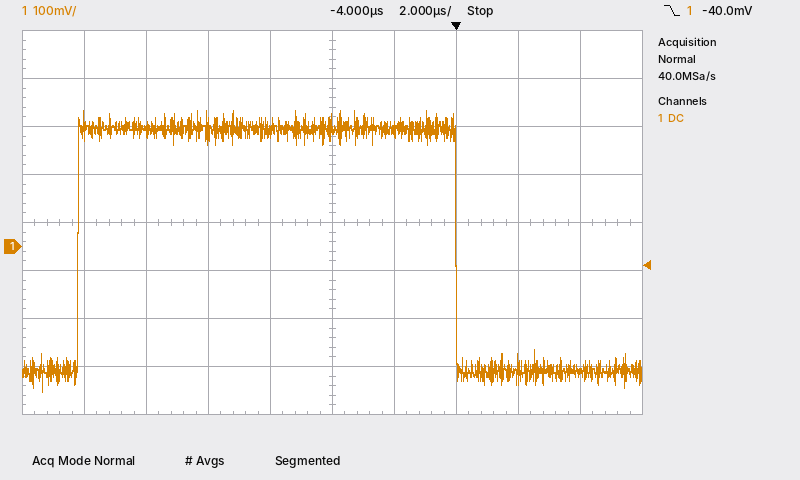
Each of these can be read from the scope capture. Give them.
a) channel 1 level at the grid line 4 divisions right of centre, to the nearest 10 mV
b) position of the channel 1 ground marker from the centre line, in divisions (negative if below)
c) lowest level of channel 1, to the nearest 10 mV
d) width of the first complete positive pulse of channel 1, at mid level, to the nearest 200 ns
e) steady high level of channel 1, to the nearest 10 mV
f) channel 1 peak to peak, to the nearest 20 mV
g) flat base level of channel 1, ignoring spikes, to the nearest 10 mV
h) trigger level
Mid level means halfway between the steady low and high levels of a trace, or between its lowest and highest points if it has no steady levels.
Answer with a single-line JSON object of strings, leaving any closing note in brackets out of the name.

{"channel 1 level at the grid line 4 divisions right of centre, to the nearest 10 mV": "-260 mV", "position of the channel 1 ground marker from the centre line, in divisions": "-0.5 div", "lowest level of channel 1, to the nearest 10 mV": "-300 mV", "width of the first complete positive pulse of channel 1, at mid level, to the nearest 200 ns": "12.2 µs", "steady high level of channel 1, to the nearest 10 mV": "250 mV", "channel 1 peak to peak, to the nearest 20 mV": "580 mV", "flat base level of channel 1, ignoring spikes, to the nearest 10 mV": "-260 mV", "trigger level": "-40.0 mV"}
